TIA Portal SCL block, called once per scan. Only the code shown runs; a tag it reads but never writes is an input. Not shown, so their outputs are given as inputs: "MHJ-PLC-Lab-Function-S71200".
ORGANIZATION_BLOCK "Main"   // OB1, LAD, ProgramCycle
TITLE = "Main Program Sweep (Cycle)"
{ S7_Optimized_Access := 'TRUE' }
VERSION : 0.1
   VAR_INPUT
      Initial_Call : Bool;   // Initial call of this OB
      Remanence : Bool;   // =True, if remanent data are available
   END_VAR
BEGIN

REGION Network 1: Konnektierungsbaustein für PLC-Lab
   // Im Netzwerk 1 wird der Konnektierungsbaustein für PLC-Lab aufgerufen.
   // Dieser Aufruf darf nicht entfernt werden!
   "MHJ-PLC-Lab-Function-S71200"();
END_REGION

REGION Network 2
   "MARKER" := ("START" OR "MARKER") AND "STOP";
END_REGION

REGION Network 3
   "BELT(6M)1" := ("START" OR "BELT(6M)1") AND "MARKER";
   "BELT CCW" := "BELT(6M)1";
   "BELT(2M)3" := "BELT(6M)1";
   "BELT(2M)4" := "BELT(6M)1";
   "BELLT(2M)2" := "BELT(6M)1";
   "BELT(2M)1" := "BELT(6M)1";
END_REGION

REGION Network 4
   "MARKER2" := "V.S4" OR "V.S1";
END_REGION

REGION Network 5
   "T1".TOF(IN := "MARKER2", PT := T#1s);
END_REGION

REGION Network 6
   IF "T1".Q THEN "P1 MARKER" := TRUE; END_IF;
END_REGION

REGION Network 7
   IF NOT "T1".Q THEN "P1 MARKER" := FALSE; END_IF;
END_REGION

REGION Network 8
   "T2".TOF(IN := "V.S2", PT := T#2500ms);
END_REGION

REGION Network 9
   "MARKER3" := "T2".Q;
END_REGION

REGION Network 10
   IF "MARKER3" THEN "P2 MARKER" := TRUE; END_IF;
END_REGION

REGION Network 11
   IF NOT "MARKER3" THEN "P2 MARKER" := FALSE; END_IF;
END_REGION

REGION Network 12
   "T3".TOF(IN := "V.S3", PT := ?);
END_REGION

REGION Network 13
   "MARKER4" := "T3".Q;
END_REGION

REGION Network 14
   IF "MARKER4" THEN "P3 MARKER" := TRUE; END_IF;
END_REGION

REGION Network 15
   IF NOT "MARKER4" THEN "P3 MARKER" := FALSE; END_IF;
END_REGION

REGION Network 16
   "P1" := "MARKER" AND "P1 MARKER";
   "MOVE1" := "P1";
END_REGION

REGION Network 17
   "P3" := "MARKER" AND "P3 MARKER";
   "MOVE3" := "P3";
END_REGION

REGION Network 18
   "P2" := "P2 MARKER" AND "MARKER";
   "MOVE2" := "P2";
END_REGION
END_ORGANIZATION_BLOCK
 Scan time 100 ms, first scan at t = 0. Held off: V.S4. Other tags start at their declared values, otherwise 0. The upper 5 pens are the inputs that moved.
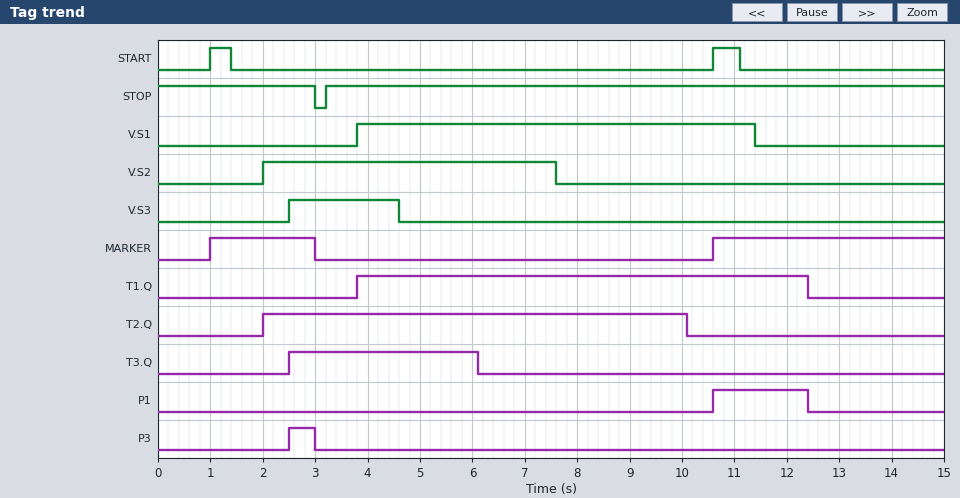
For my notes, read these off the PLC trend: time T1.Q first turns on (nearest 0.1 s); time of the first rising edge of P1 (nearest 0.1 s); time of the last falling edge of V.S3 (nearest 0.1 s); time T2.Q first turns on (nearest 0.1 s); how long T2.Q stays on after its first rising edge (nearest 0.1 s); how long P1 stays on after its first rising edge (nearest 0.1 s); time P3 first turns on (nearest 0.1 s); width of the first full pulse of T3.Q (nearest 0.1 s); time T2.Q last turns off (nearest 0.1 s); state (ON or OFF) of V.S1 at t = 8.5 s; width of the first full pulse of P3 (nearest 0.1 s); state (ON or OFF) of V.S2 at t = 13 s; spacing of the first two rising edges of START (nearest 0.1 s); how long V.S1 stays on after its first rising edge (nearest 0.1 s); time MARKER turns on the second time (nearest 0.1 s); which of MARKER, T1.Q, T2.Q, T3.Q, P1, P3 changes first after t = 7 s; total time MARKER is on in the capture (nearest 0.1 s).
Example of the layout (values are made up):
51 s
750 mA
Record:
3.8 s
10.6 s
4.6 s
2.0 s
8.1 s
1.8 s
2.5 s
3.6 s
10.1 s
ON
0.5 s
OFF
9.6 s
7.6 s
10.6 s
T2.Q
6.4 s
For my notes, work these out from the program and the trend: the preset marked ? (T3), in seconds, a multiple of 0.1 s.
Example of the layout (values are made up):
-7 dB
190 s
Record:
1.5 s
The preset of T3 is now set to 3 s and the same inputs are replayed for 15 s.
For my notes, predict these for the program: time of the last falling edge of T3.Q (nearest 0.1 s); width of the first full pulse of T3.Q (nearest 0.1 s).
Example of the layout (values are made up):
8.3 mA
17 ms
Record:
7.6 s
5.1 s
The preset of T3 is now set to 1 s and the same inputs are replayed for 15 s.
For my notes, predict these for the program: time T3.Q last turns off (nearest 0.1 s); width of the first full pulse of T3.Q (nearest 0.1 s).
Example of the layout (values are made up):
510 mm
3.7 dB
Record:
5.6 s
3.1 s
